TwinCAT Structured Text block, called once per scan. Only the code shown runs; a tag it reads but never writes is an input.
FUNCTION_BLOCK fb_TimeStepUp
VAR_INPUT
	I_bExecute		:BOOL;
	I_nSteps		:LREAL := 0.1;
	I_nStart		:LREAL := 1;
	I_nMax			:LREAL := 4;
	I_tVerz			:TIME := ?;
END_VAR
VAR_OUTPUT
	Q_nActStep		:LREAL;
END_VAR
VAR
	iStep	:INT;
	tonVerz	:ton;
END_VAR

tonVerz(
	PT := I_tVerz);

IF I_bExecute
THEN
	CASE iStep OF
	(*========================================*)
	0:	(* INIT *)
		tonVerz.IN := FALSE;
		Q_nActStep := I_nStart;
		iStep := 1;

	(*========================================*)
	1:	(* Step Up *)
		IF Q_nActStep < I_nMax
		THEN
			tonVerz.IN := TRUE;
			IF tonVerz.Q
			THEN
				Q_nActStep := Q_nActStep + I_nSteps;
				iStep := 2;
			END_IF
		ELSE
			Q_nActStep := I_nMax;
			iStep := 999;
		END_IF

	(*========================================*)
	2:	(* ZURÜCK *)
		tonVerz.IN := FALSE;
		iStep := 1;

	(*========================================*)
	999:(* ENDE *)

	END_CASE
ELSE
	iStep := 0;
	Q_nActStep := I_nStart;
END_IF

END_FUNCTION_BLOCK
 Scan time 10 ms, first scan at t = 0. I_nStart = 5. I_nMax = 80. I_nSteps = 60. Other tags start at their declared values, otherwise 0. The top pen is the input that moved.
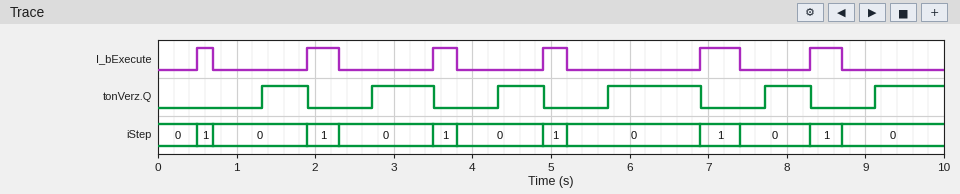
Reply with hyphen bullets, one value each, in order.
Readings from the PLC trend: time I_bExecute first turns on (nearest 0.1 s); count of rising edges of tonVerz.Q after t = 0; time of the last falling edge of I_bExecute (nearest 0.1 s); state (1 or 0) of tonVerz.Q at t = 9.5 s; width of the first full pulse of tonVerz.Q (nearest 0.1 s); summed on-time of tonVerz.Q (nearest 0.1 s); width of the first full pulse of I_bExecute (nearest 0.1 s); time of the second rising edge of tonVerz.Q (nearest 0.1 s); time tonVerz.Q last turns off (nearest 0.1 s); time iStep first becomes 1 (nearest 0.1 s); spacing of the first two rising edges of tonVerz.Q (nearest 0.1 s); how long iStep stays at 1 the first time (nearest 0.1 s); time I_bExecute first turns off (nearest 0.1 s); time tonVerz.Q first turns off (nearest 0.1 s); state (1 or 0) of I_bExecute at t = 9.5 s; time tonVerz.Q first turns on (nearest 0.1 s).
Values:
- 0.5 s
- 6
- 8.7 s
- 1
- 0.6 s
- 4.6 s
- 0.2 s
- 2.7 s
- 8.3 s
- 0.5 s
- 1.4 s
- 0.2 s
- 0.7 s
- 1.9 s
- 0
- 1.3 s
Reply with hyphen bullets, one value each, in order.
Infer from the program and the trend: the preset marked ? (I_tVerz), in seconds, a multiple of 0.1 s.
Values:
- 0.8 s
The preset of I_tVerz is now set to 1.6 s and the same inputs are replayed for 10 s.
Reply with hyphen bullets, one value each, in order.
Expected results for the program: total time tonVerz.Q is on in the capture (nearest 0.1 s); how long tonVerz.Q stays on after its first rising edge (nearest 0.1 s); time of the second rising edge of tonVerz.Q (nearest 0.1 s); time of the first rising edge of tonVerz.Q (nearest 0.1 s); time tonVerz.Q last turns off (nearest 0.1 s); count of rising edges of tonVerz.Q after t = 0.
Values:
- 0.5 s
- 0.4 s
- 9.9 s
- 6.5 s
- 6.9 s
- 2
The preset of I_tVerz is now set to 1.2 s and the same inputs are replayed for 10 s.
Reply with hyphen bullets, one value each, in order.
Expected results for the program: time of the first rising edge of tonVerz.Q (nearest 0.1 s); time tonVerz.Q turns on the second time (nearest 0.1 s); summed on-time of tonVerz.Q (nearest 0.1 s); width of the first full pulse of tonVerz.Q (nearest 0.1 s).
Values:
- 1.7 s
- 3.1 s
- 2.2 s
- 0.2 s
